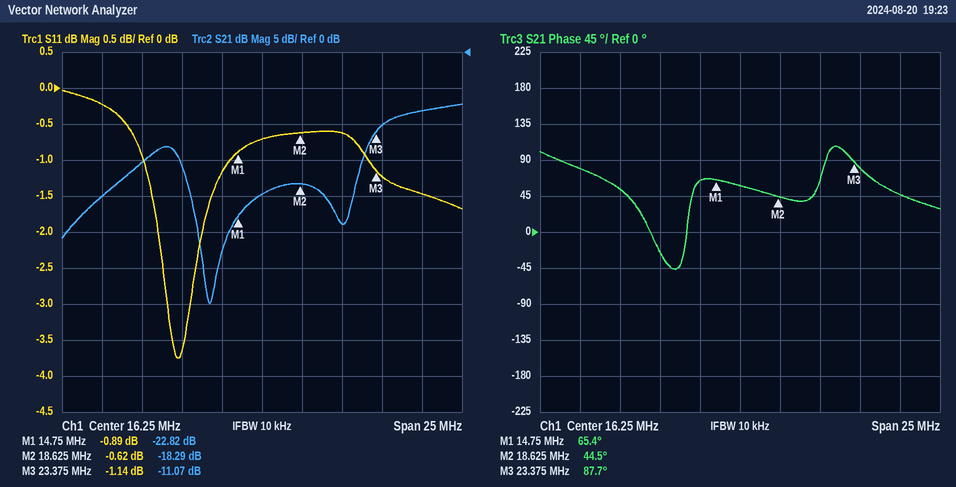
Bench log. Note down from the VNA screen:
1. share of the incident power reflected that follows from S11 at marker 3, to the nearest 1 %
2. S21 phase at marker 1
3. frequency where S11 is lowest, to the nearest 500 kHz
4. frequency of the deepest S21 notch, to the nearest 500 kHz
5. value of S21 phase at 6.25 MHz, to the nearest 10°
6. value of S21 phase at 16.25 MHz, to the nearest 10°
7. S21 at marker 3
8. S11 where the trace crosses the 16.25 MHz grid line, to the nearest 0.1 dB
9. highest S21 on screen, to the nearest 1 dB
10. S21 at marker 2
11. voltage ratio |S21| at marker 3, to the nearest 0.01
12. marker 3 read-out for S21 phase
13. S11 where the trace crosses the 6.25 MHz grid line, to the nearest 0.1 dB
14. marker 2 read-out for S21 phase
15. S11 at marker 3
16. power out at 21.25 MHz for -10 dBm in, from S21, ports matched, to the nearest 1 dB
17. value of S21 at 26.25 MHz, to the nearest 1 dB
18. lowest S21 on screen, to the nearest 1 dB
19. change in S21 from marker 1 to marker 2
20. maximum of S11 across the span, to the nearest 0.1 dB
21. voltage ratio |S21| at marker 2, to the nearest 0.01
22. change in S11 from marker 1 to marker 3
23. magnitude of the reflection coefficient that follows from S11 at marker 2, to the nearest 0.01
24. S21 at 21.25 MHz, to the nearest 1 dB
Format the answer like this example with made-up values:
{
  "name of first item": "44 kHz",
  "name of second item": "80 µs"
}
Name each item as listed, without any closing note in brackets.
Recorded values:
{
  "share of the incident power reflected that follows from S11 at marker 3, to the nearest 1 %": "77 %",
  "S21 phase at marker 1": "65.4°",
  "frequency where S11 is lowest, to the nearest 500 kHz": "11.0 MHz",
  "frequency of the deepest S21 notch, to the nearest 500 kHz": "13.0 MHz",
  "value of S21 phase at 6.25 MHz, to the nearest 10°": "80°",
  "value of S21 phase at 16.25 MHz, to the nearest 10°": "60°",
  "S21 at marker 3": "-11.07 dB",
  "S11 where the trace crosses the 16.25 MHz grid line, to the nearest 0.1 dB": "-0.7 dB",
  "highest S21 on screen, to the nearest 1 dB": "-7 dB",
  "S21 at marker 2": "-18.29 dB",
  "voltage ratio |S21| at marker 3, to the nearest 0.01": "0.28",
  "marker 3 read-out for S21 phase": "87.7°",
  "S11 where the trace crosses the 6.25 MHz grid line, to the nearest 0.1 dB": "-0.2 dB",
  "marker 2 read-out for S21 phase": "44.5°",
  "S11 at marker 3": "-1.14 dB",
  "power out at 21.25 MHz for -10 dBm in, from S21, ports matched, to the nearest 1 dB": "-34 dBm",
  "value of S21 at 26.25 MHz, to the nearest 1 dB": "-8 dB",
  "lowest S21 on screen, to the nearest 1 dB": "-35 dB",
  "change in S21 from marker 1 to marker 2": "4.53 dB",
  "maximum of S11 across the span, to the nearest 0.1 dB": "0.0 dB",
  "voltage ratio |S21| at marker 2, to the nearest 0.01": "0.12",
  "change in S11 from marker 1 to marker 3": "-0.25 dB",
  "magnitude of the reflection coefficient that follows from S11 at marker 2, to the nearest 0.01": "0.93",
  "S21 at 21.25 MHz, to the nearest 1 dB": "-24 dB"
}
